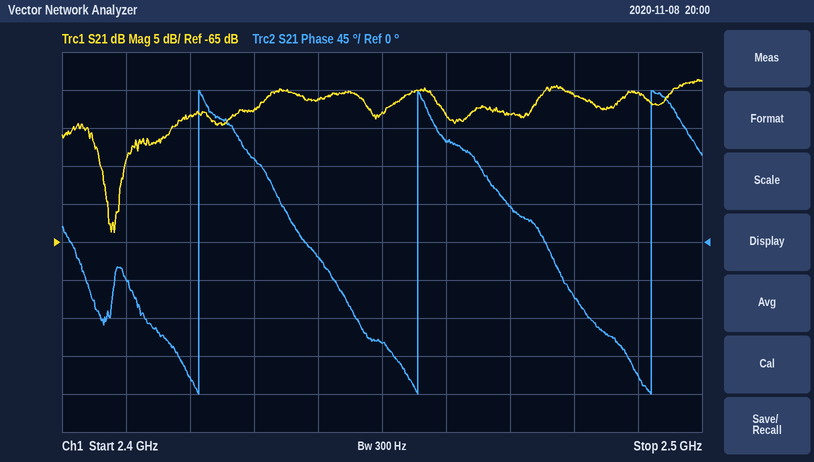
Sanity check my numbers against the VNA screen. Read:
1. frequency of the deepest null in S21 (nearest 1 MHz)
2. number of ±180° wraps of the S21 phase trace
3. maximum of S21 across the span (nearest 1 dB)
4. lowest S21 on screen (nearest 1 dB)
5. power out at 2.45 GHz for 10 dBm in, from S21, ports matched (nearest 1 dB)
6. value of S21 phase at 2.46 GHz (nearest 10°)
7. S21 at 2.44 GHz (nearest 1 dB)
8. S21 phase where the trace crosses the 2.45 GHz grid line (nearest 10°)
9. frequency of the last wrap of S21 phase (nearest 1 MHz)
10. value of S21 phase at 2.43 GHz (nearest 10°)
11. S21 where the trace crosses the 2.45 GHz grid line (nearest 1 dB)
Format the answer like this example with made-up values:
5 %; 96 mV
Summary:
2.408 GHz; 3; -44 dB; -64 dB; -38 dBm; 120°; -46 dB; -120°; 2.492 GHz; 100°; -48 dB
